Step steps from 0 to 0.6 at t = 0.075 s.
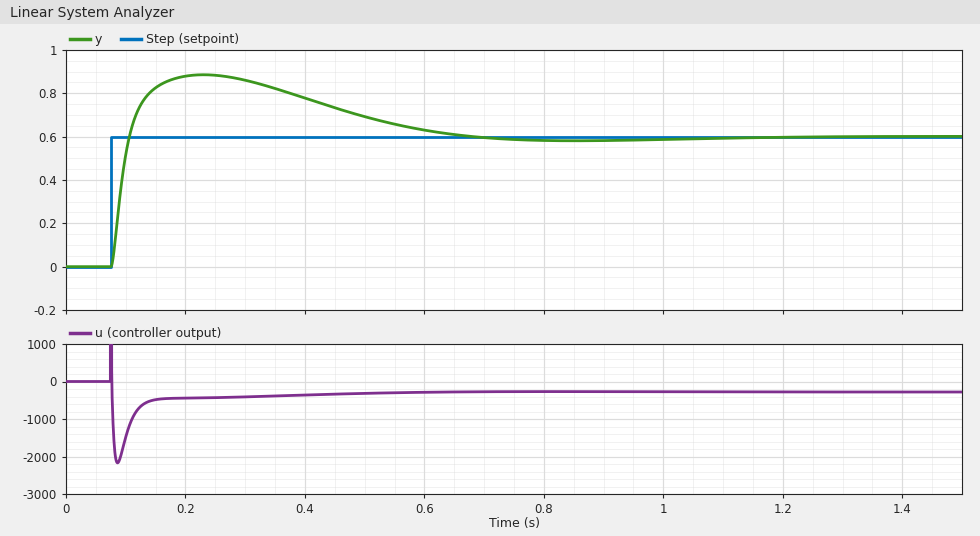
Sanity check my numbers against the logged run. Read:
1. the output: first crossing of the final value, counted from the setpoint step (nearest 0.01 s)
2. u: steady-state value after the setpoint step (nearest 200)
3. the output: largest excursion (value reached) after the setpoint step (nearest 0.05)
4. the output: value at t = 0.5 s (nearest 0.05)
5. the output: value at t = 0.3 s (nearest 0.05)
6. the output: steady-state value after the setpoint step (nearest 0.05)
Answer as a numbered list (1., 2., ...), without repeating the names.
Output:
1. 0.03 s
2. -200
3. 0.90
4. 0.70
5. 0.85
6. 0.60
